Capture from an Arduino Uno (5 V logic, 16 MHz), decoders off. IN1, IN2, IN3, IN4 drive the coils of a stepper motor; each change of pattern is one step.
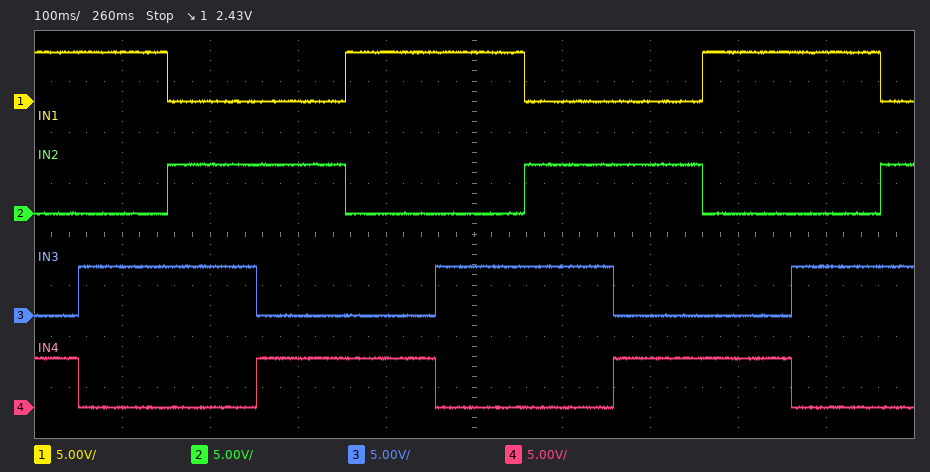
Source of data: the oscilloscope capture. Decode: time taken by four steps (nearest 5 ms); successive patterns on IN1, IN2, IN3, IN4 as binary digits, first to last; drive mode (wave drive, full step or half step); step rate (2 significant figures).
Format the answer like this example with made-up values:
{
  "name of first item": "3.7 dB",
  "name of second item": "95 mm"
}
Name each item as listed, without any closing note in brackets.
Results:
{
  "time taken by four steps": "405 ms",
  "successive patterns on IN1, IN2, IN3, IN4 as binary digits, first to last": "1001 1010 0110 0101 1001 1010 0110 0101 1001 1010 0110",
  "drive mode": "full step",
  "step rate": "9.9 steps/s"
}
